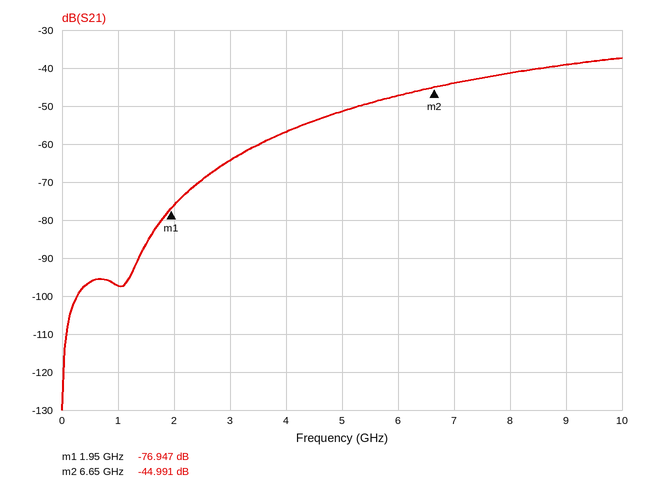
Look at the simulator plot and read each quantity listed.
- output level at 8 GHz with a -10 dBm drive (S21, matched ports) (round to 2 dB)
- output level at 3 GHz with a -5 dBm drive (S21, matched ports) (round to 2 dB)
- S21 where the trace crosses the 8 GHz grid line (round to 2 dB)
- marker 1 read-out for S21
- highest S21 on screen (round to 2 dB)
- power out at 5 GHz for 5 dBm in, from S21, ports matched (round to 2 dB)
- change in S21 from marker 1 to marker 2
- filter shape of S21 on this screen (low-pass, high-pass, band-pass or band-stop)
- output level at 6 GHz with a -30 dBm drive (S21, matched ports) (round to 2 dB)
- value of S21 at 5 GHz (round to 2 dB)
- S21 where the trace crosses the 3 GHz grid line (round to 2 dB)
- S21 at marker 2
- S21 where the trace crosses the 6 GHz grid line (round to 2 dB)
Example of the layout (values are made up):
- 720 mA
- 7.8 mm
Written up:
- -52 dBm
- -70 dBm
- -42 dB
- -76.947 dB
- -38 dB
- -46 dBm
- 31.956 dB
- high-pass
- -78 dBm
- -52 dB
- -64 dB
- -44.991 dB
- -48 dB
